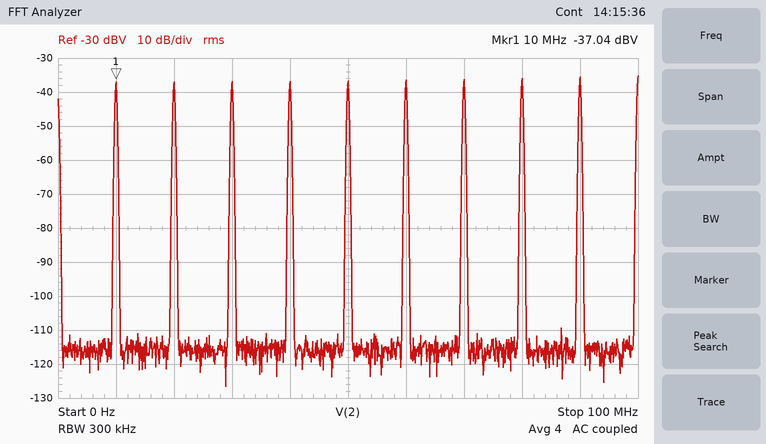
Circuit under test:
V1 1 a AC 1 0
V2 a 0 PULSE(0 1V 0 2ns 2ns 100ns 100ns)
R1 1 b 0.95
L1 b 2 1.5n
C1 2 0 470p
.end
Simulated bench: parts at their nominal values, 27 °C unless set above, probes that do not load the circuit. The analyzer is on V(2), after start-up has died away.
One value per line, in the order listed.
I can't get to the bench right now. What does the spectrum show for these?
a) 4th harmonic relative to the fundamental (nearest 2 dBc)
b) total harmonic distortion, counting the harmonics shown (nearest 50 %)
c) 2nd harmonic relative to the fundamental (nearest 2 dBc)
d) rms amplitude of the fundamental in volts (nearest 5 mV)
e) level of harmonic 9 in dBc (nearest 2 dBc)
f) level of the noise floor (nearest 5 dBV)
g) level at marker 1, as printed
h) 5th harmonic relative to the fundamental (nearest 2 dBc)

0 dBc
300 %
0 dBc
15 mV
2 dBc
-115 dBV
-37.04 dBV
0 dBc
